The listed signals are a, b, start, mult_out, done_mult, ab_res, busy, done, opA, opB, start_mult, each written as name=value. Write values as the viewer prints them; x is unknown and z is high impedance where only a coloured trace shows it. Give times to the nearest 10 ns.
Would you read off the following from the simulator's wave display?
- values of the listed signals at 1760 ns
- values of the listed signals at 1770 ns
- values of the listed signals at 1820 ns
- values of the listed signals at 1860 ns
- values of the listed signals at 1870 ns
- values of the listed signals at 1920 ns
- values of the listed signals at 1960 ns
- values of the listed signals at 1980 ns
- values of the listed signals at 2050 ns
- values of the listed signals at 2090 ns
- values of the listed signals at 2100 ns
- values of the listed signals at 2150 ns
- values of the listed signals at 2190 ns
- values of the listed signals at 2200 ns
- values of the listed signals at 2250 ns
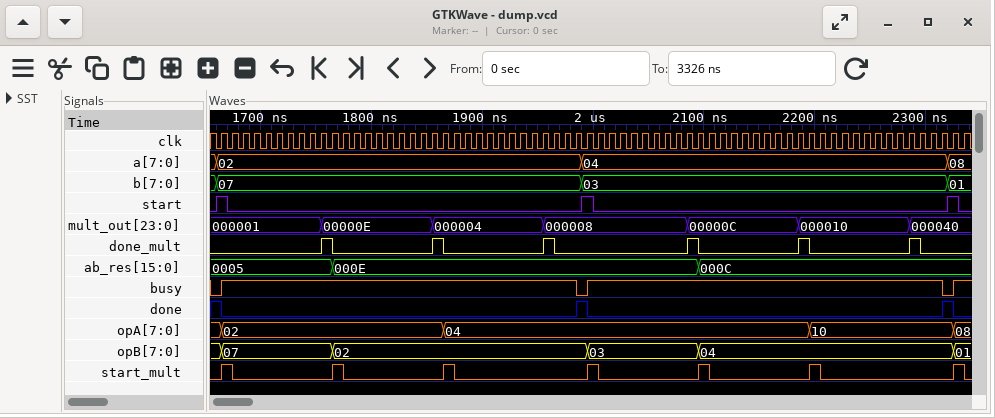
a=02, b=07, start=0, mult_out=00000E, done_mult=1, ab_res=0005, busy=1, done=0, opA=02, opB=07, start_mult=0
a=02, b=07, start=0, mult_out=00000E, done_mult=0, ab_res=000E, busy=1, done=0, opA=02, opB=02, start_mult=1
a=02, b=07, start=0, mult_out=00000E, done_mult=0, ab_res=000E, busy=1, done=0, opA=02, opB=02, start_mult=0
a=02, b=07, start=0, mult_out=000004, done_mult=1, ab_res=000E, busy=1, done=0, opA=02, opB=02, start_mult=0
a=02, b=07, start=0, mult_out=000004, done_mult=0, ab_res=000E, busy=1, done=0, opA=04, opB=02, start_mult=1
a=02, b=07, start=0, mult_out=000004, done_mult=0, ab_res=000E, busy=1, done=0, opA=04, opB=02, start_mult=0
a=02, b=07, start=0, mult_out=000008, done_mult=1, ab_res=000E, busy=1, done=0, opA=04, opB=02, start_mult=0
a=02, b=07, start=0, mult_out=000008, done_mult=0, ab_res=000E, busy=1, done=0, opA=04, opB=02, start_mult=0
a=04, b=03, start=0, mult_out=000008, done_mult=0, ab_res=000E, busy=1, done=0, opA=04, opB=03, start_mult=0
a=04, b=03, start=0, mult_out=00000C, done_mult=1, ab_res=000E, busy=1, done=0, opA=04, opB=03, start_mult=0
a=04, b=03, start=0, mult_out=00000C, done_mult=0, ab_res=000C, busy=1, done=0, opA=04, opB=04, start_mult=1
a=04, b=03, start=0, mult_out=00000C, done_mult=0, ab_res=000C, busy=1, done=0, opA=04, opB=04, start_mult=0
a=04, b=03, start=0, mult_out=000010, done_mult=1, ab_res=000C, busy=1, done=0, opA=04, opB=04, start_mult=0
a=04, b=03, start=0, mult_out=000010, done_mult=0, ab_res=000C, busy=1, done=0, opA=10, opB=04, start_mult=1
a=04, b=03, start=0, mult_out=000010, done_mult=0, ab_res=000C, busy=1, done=0, opA=10, opB=04, start_mult=0
